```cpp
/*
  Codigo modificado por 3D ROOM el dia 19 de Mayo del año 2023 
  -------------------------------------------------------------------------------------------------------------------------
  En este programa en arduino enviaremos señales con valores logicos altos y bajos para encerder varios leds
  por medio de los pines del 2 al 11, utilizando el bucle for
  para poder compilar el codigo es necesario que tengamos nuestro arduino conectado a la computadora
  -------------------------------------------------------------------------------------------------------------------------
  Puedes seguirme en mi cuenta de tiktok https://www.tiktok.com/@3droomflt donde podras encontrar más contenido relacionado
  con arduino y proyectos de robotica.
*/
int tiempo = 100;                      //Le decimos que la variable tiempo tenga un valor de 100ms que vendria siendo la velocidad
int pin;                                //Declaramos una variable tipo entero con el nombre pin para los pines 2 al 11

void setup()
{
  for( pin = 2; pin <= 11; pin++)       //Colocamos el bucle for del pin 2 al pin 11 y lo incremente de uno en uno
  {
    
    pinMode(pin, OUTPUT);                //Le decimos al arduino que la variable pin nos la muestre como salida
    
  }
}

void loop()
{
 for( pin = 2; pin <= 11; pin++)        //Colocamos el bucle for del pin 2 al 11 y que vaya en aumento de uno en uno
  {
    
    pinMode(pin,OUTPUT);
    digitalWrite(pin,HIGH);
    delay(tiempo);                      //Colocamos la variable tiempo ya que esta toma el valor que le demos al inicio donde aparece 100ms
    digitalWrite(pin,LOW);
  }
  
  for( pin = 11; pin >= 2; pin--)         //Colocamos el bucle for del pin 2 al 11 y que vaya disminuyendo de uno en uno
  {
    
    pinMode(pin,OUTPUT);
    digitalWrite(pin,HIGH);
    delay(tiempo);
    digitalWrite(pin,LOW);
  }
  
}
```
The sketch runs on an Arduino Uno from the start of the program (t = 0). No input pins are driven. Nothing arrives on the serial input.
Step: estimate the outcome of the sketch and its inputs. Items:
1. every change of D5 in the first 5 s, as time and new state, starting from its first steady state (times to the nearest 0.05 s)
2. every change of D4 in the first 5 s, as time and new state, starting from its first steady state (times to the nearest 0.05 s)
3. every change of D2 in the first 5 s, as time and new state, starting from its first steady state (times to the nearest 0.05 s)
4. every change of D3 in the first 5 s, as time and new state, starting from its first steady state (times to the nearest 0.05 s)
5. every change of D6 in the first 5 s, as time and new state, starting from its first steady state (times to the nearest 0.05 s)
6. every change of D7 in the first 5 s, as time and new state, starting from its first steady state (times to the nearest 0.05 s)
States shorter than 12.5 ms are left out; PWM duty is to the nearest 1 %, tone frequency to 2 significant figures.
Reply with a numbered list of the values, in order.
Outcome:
1. 0 s low; 0.3 s high; 0.4 s low; 1.6 s high; 1.7 s low; 2.3 s high; 2.4 s low; 3.6 s high; 3.7 s low; 4.3 s high; 4.4 s low
2. 0 s low; 0.2 s high; 0.3 s low; 1.7 s high; 1.8 s low; 2.2 s high; 2.3 s low; 3.7 s high; 3.8 s low; 4.2 s high; 4.3 s low
3. 0 s high; 0.1 s low; 1.9 s high; 2.1 s low; 3.9 s high; 4.1 s low
4. 0 s low; 0.1 s high; 0.2 s low; 1.8 s high; 1.9 s low; 2.1 s high; 2.2 s low; 3.8 s high; 3.9 s low; 4.1 s high; 4.2 s low
5. 0 s low; 0.4 s high; 0.5 s low; 1.5 s high; 1.6 s low; 2.4 s high; 2.5 s low; 3.5 s high; 3.6 s low; 4.4 s high; 4.5 s low
6. 0 s low; 0.5 s high; 0.6 s low; 1.4 s high; 1.5 s low; 2.5 s high; 2.6 s low; 3.4 s high; 3.5 s low; 4.5 s high; 4.6 s low
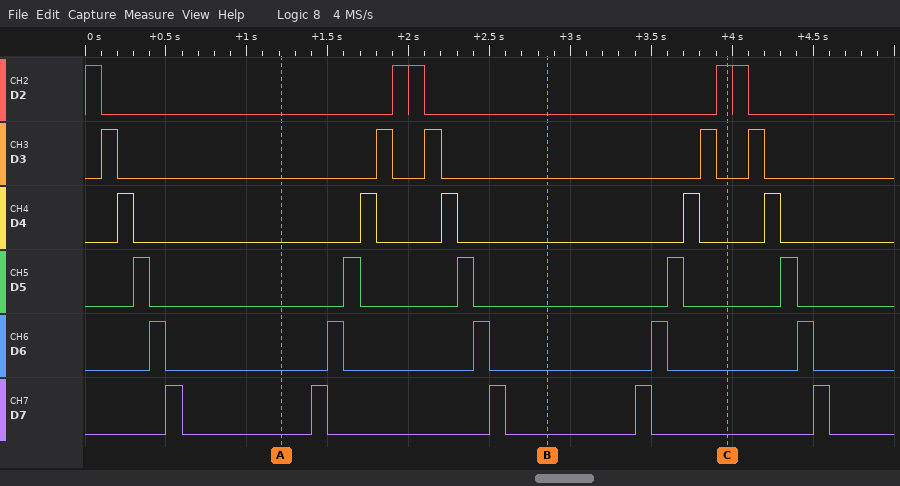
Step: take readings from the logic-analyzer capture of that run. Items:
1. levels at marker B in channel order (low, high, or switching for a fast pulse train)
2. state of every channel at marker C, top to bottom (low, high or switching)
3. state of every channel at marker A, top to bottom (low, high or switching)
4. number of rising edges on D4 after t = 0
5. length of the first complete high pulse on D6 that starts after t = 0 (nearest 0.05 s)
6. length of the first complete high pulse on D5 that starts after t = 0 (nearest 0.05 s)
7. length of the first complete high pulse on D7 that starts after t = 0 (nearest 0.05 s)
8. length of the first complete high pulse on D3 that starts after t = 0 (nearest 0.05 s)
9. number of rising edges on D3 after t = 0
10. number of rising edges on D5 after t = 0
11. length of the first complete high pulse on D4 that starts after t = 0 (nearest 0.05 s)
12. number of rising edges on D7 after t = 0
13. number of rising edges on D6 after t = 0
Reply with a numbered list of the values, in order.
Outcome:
1. D2 low, D3 low, D4 low, D5 low, D6 low, D7 low
2. D2 high, D3 low, D4 low, D5 low, D6 low, D7 low
3. D2 low, D3 low, D4 low, D5 low, D6 low, D7 low
4. 5
5. 0.10 s
6. 0.10 s
7. 0.10 s
8. 0.10 s
9. 5
10. 5
11. 0.10 s
12. 5
13. 5
